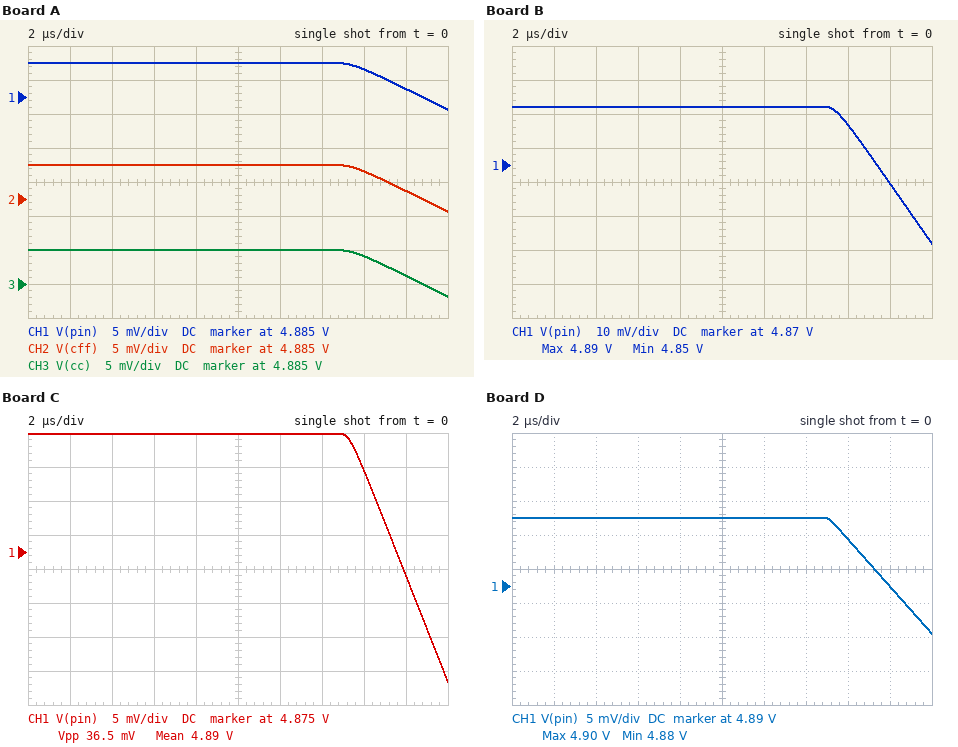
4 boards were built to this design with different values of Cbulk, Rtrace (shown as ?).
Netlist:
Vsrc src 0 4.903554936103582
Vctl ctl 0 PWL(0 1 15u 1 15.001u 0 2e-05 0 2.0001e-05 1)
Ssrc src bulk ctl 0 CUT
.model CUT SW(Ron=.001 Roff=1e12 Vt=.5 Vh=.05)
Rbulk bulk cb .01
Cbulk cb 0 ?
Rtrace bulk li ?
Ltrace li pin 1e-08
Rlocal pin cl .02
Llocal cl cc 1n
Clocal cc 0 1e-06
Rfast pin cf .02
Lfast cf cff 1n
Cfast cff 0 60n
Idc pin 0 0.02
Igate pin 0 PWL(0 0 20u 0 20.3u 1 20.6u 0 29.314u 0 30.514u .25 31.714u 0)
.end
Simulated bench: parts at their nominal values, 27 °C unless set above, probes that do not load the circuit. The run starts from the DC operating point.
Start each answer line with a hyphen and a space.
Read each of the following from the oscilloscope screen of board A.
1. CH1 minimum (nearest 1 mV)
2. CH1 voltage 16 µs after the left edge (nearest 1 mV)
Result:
- 4.883 V
- 4.889 V
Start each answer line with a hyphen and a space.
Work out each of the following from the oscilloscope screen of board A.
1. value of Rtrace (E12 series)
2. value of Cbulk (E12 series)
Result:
- 0.68 Ω
- 12 µF
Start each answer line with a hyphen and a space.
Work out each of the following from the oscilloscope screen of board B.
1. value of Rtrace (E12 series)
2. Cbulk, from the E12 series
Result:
- 0.82 Ω
- 1.2 µF
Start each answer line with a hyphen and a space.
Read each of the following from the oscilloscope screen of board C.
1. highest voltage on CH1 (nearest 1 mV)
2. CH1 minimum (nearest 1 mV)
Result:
- 4.892 V
- 4.856 V
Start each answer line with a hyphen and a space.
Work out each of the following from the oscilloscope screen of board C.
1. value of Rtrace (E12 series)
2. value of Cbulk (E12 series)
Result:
- 0.56 Ω
- 1.5 µF
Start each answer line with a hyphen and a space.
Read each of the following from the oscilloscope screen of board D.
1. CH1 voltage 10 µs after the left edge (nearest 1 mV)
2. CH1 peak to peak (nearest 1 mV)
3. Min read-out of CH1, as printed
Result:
- 4.900 V
- 17 mV
- 4.88 V
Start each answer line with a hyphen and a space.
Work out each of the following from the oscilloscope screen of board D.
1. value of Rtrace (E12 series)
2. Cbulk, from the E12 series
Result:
- 0.18 Ω
- 4.7 µF
